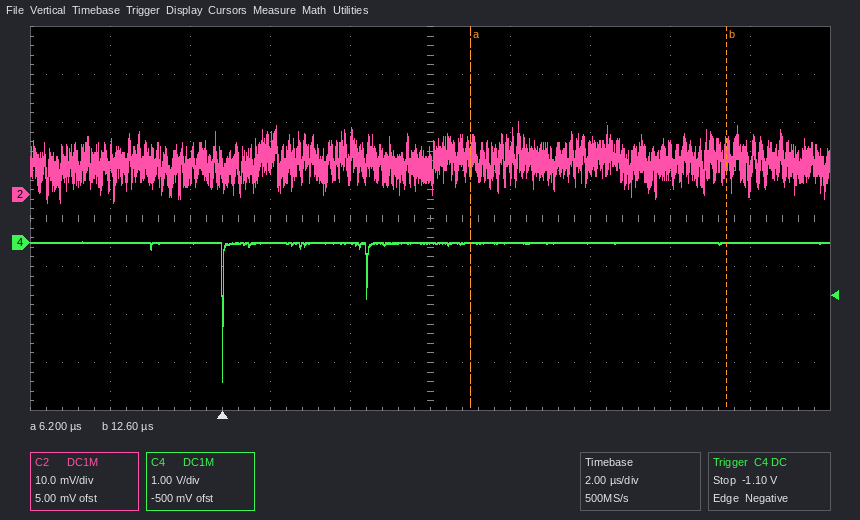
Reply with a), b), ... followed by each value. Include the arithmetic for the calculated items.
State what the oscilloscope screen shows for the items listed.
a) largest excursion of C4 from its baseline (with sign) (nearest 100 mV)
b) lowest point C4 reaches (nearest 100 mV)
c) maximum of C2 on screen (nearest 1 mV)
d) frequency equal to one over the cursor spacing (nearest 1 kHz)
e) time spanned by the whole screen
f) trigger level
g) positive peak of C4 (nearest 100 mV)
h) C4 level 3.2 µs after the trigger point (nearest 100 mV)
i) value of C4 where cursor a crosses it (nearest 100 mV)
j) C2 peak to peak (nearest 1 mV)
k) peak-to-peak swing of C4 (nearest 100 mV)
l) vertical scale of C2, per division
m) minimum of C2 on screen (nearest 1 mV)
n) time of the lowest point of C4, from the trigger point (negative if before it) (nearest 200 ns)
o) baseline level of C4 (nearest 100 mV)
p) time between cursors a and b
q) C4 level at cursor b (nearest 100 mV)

a) -2.9 V − (0.0 V) = -2.9 V
b) -2.9 V
c) 15 mV
d) 1 / 6.4 µs ≈ 156 kHz
e) 20 µs
f) -1.10 V
g) 0.0 V
h) 0.0 V
i) 0.0 V
j) 15 mV − (-2 mV) = 17 mV
k) 0.0 V − (-2.9 V) = 2.9 V
l) 10 mV
m) -2 mV
n) 0.0 µs
o) 0.0 V
p) 12.6 µs − (6.2 µs) = 6.4 µs
q) 0.0 V
